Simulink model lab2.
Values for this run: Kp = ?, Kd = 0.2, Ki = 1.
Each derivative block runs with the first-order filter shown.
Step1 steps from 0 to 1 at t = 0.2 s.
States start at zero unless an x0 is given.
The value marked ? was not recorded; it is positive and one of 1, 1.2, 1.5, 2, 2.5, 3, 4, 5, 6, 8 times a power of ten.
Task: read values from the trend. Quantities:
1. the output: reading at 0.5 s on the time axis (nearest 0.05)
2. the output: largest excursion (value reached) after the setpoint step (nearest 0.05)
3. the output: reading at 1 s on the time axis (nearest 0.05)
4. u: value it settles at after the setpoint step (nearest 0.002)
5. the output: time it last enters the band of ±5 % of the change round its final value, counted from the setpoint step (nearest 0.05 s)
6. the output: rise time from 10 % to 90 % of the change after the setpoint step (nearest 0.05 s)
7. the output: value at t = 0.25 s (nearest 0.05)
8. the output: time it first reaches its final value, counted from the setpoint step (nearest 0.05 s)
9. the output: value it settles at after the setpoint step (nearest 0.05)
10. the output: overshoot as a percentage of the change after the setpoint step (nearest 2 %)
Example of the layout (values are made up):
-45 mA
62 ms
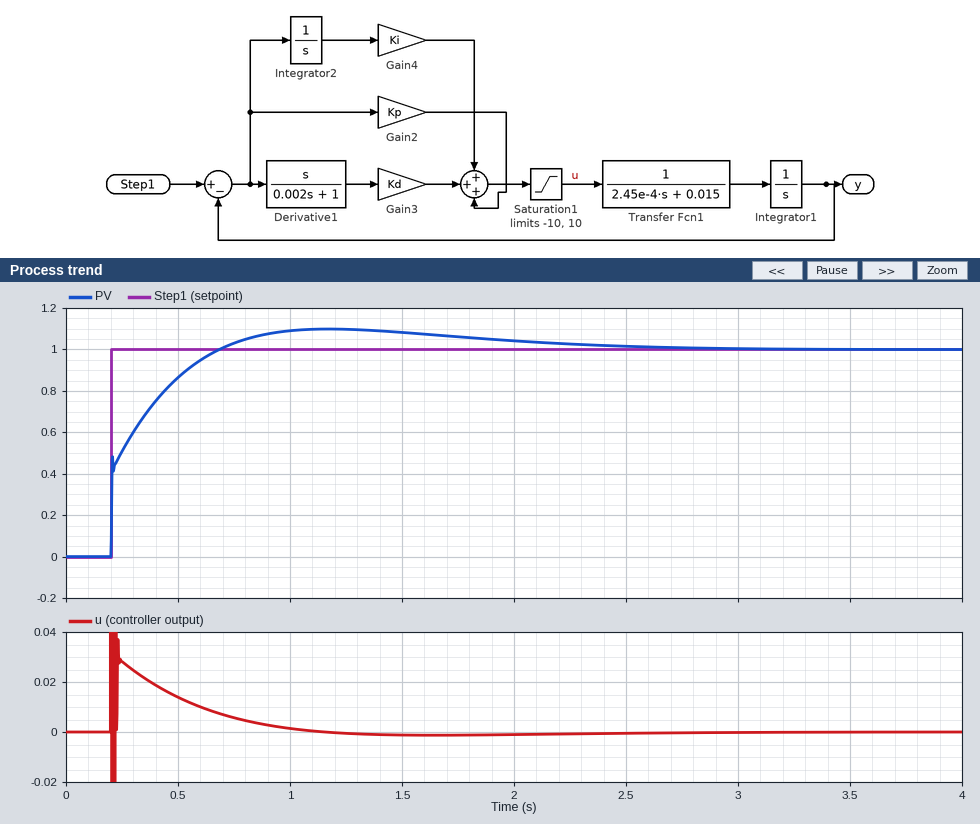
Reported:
0.85
1.10
1.10
0.000
1.70 s
0.35 s
0.50
0.50 s
1.00
10 %
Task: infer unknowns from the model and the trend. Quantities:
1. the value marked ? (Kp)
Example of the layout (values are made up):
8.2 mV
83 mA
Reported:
0.8
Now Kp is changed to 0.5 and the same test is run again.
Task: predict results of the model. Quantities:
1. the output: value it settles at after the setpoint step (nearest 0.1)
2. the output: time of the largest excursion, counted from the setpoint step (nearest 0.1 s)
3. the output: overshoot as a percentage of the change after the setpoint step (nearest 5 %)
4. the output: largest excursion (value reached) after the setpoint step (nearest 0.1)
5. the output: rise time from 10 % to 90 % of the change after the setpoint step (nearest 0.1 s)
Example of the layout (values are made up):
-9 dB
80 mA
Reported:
1.0
1.1 s
15 %
1.2
0.4 s
